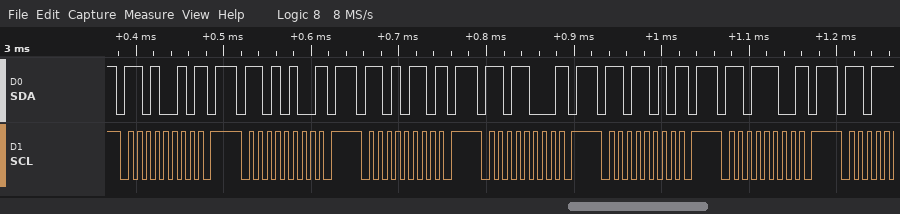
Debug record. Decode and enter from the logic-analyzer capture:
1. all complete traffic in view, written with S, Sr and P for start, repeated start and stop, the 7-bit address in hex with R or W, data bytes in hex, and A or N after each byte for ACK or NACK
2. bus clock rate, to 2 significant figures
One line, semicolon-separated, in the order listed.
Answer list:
S 69W N P S 6AW N P S 6BW N P S 6CW N P S 6DW N P S 6EW N P; 100 kHz
